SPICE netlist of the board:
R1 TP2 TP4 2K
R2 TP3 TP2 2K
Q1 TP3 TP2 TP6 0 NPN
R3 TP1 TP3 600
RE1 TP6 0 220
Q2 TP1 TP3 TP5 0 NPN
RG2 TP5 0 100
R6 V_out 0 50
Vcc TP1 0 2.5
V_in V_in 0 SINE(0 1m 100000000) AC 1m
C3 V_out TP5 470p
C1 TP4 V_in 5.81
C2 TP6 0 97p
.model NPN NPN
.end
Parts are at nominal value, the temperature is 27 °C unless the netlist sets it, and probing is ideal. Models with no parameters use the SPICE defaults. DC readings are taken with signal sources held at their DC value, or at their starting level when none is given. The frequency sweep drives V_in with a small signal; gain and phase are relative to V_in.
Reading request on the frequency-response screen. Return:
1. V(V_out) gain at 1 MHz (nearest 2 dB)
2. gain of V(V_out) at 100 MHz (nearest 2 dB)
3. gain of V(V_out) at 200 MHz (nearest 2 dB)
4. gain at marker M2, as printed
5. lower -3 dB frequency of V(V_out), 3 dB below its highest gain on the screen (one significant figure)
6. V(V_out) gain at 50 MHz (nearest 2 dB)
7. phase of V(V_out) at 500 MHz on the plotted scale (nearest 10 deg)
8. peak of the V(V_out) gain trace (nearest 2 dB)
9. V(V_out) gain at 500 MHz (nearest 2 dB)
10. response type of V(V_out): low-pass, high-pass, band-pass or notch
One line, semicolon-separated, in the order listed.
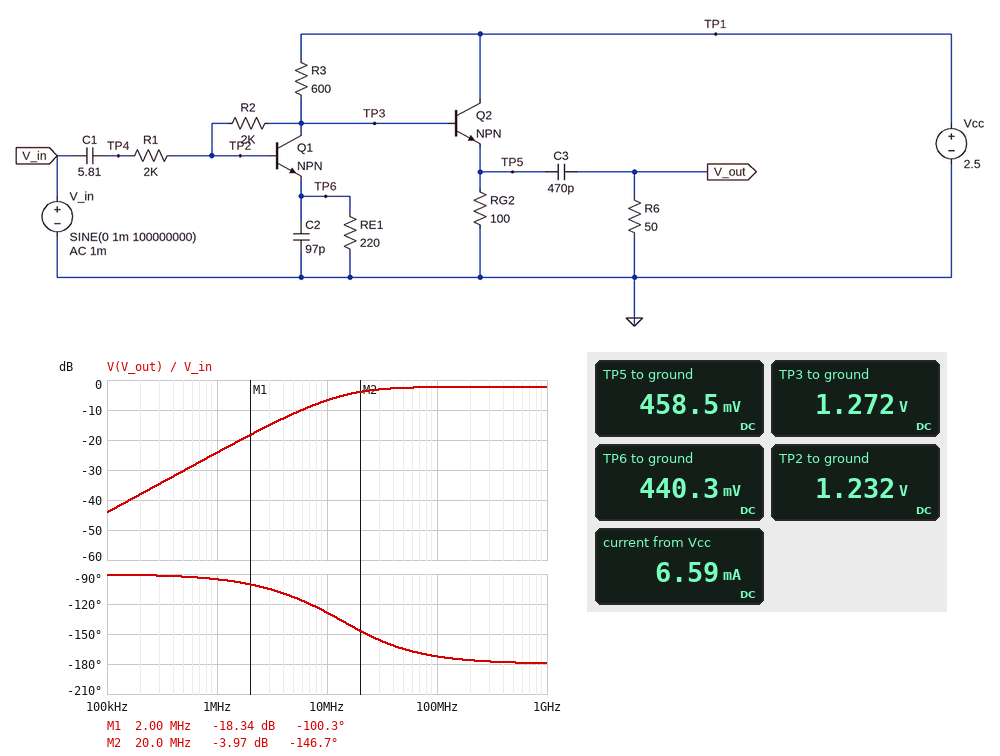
-24 dB; -2 dB; -2 dB; -3.97 dB; 10 MHz; -2 dB; -180 deg; -2 dB; -2 dB; high-pass
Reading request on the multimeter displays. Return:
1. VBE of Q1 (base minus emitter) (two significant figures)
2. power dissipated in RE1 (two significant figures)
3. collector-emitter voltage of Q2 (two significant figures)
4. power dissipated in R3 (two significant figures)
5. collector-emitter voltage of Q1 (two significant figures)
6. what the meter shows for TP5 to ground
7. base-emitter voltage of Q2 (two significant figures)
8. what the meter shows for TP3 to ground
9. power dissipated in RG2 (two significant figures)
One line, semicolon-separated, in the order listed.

790 mV; 880 µW; 2.0 V; 2.5 mW; 830 mV; 458.5 mV; 810 mV; 1.272 V; 2.1 mW
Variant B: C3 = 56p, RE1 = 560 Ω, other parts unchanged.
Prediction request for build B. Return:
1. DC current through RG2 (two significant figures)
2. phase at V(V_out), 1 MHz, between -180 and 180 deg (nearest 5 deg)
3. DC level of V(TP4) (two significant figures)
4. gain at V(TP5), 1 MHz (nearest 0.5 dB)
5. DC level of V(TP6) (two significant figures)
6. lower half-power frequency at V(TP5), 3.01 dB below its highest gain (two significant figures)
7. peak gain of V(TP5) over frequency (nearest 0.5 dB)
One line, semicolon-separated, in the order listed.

7.8 mA; -70 deg; 1.6 V; -13.0 dB; 790 mV; 7.6 MHz; -2.0 dB
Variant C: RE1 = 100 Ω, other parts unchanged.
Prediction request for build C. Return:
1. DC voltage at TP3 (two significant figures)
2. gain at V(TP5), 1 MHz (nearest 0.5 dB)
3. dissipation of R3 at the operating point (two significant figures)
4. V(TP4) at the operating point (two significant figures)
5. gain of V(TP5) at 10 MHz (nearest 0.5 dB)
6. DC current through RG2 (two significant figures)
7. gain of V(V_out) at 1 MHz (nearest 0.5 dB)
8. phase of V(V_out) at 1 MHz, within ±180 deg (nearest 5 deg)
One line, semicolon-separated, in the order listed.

1.1 V; -5.0 dB; 3.4 mW; 1.0 V; -5.0 dB; 2.8 mA; -21.5 dB; -100 deg
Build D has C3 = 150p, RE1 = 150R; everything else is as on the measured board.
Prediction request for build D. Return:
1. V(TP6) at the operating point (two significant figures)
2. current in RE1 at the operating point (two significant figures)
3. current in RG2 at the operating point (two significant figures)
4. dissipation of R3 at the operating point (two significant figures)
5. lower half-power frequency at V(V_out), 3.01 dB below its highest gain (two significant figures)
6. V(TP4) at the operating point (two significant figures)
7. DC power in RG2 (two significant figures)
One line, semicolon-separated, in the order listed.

330 mV; 2.2 mA; 3.6 mA; 3.0 mW; 25 MHz; 1.1 V; 1.3 mW
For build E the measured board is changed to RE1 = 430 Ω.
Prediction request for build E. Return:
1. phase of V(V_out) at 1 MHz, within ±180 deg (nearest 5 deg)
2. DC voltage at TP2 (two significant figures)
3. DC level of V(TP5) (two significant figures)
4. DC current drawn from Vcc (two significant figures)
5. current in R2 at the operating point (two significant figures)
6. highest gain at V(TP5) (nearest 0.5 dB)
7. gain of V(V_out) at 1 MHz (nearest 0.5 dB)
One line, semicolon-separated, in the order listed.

-85 deg; 1.5 V; 680 mV; 8.4 mA; 16 µA; -2.0 dB; -28.0 dB
